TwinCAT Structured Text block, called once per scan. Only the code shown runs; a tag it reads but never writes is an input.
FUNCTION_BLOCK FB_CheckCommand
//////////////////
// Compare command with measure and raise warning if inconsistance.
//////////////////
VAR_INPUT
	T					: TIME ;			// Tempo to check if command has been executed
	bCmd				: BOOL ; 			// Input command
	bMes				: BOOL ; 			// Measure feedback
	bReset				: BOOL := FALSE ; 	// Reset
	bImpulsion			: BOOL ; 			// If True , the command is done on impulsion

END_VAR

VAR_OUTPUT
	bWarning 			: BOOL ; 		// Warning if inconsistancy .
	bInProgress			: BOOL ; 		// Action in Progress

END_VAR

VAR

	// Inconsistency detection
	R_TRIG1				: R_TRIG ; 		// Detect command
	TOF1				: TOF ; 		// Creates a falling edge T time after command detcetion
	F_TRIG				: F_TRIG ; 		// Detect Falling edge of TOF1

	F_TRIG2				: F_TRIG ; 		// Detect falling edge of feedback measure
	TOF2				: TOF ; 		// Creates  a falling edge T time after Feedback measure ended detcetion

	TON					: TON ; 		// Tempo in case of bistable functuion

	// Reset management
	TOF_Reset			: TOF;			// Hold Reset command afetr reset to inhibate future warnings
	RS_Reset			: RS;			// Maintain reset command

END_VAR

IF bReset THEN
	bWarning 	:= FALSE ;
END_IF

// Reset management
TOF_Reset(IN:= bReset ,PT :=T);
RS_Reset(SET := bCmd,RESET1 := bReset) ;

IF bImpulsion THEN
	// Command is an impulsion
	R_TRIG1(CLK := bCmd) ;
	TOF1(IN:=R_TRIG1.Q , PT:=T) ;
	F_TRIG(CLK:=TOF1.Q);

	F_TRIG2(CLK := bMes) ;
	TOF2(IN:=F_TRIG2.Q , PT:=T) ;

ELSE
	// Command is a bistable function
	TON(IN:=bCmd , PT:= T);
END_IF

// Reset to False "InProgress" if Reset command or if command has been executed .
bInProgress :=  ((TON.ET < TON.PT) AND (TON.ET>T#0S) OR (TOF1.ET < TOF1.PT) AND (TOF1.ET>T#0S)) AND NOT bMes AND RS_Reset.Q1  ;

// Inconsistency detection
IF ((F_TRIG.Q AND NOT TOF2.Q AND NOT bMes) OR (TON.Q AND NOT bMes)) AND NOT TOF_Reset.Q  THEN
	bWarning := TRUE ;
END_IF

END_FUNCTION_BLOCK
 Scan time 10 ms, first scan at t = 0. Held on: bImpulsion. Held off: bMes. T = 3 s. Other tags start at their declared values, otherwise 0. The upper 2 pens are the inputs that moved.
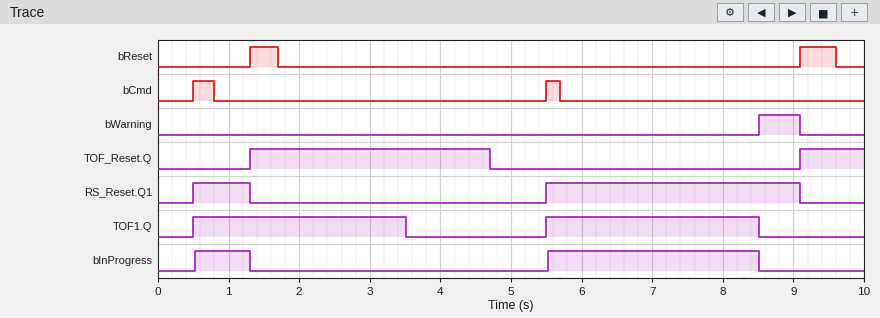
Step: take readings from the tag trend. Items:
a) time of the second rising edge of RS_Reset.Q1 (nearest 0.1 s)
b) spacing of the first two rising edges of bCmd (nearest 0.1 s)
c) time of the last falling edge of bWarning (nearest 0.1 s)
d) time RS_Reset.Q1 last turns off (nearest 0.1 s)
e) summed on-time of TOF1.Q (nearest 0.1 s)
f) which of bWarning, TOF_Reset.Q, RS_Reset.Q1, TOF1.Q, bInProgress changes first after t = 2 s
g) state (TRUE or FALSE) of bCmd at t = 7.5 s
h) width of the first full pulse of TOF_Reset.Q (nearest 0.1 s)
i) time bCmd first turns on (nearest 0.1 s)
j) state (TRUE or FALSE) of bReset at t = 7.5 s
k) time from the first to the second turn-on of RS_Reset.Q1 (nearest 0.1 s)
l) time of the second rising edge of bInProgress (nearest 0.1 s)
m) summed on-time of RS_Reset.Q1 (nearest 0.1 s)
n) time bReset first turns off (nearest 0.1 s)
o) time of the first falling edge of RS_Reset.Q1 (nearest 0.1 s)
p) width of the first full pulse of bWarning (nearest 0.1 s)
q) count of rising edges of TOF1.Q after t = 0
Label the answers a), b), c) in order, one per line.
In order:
a) 5.5 s
b) 5.0 s
c) 9.1 s
d) 9.1 s
e) 6.0 s
f) TOF1.Q
g) FALSE
h) 3.4 s
i) 0.5 s
j) FALSE
k) 5.0 s
l) 5.5 s
m) 4.4 s
n) 1.7 s
o) 1.3 s
p) 0.6 s
q) 2
